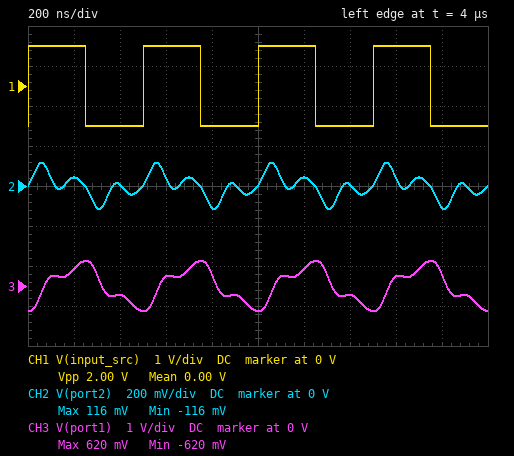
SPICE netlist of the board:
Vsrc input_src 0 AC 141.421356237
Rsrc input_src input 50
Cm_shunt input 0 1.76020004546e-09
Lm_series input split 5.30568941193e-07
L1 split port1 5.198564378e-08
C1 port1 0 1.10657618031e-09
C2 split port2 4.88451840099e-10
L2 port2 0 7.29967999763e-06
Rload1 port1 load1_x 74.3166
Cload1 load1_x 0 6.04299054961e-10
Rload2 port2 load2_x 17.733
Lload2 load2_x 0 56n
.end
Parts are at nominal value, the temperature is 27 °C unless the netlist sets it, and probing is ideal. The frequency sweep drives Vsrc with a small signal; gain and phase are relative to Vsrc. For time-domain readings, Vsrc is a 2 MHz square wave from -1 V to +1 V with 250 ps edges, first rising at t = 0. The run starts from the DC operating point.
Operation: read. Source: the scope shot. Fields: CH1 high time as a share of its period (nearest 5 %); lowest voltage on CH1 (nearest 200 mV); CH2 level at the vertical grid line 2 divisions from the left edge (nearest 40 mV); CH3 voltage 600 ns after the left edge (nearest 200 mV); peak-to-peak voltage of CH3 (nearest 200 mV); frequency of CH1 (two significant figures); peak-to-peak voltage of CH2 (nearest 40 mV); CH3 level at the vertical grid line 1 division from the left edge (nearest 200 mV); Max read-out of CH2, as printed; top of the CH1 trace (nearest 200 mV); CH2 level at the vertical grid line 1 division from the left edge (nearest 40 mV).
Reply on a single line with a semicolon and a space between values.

50 %; -1.0 V; 0 V; 200 mV; 1.2 V; 2.0 MHz; 240 mV; 400 mV; 116 mV; 1.0 V; 40 mV
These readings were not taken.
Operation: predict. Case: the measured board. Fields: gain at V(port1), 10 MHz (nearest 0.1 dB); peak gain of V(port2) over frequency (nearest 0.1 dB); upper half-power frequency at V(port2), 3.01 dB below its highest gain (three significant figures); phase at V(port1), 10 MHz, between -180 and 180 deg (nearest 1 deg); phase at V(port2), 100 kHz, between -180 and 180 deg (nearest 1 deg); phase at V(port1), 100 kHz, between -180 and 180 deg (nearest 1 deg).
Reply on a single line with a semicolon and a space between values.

-19.5 dB; -14.8 dB; 7.94 MHz; 127 deg; 158 deg; -7 deg
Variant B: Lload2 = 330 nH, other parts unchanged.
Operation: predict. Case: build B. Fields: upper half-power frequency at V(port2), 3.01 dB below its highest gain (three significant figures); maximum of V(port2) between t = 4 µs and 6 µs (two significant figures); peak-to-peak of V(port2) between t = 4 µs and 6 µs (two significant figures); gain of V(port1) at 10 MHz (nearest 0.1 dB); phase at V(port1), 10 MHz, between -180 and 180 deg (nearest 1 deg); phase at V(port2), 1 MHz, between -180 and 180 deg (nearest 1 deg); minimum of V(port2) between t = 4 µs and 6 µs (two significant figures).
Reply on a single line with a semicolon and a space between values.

7.99 MHz; 150 mV; 300 mV; -20.9 dB; 137 deg; 64 deg; -150 mV
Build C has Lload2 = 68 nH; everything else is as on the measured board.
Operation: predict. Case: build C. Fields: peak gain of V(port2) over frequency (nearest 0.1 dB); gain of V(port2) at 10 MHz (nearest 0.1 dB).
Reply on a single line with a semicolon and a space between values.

-14.7 dB; -27.1 dB
